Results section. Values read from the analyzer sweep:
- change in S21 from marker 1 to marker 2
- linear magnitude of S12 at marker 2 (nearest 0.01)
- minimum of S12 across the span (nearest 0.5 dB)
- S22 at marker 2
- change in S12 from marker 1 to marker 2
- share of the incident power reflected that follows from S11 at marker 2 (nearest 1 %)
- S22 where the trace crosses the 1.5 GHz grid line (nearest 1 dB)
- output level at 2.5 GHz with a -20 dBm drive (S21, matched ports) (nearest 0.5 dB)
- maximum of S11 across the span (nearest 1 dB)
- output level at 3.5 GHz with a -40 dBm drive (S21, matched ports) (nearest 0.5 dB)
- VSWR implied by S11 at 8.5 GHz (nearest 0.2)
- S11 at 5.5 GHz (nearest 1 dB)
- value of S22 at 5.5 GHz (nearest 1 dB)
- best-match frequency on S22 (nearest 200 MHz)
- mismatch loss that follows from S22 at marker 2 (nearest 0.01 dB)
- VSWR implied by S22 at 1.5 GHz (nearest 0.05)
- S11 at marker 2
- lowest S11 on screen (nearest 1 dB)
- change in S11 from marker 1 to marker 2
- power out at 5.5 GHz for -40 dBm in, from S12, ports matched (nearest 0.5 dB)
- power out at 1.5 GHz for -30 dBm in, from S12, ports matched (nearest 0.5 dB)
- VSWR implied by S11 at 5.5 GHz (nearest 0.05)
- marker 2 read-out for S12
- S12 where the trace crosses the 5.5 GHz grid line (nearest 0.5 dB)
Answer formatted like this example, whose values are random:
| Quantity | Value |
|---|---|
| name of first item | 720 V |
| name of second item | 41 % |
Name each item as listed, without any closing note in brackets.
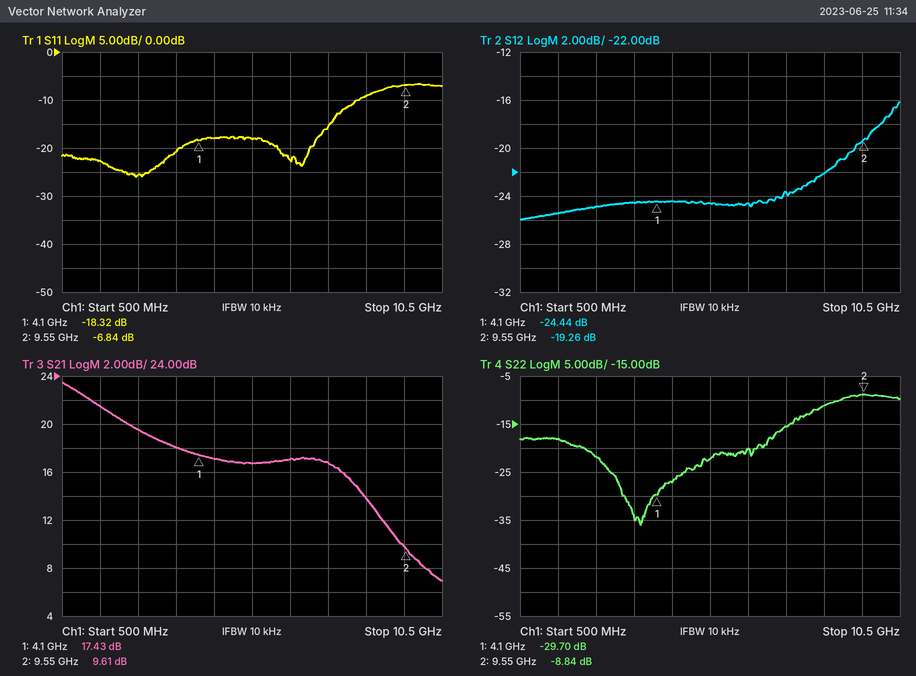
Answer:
| Quantity | Value |
|---|---|
| change in S21 from marker 1 to marker 2 | -7.82 dB |
| linear magnitude of S12 at marker 2 | 0.11 |
| minimum of S12 across the span | -26.0 dB |
| S22 at marker 2 | -8.84 dB |
| change in S12 from marker 1 to marker 2 | 5.18 dB |
| share of the incident power reflected that follows from S11 at marker 2 | 21 % |
| S22 where the trace crosses the 1.5 GHz grid line | -18 dB |
| output level at 2.5 GHz with a -20 dBm drive (S21, matched ports) | -0.5 dBm |
| maximum of S11 across the span | -7 dB |
| output level at 3.5 GHz with a -40 dBm drive (S21, matched ports) | -22.0 dBm |
| VSWR implied by S11 at 8.5 GHz | 2.0 |
| S11 at 5.5 GHz | -18 dB |
| value of S22 at 5.5 GHz | -22 dB |
| best-match frequency on S22 | 3.6 GHz |
| mismatch loss that follows from S22 at marker 2 | 0.61 dB |
| VSWR implied by S22 at 1.5 GHz | 1.30 |
| S11 at marker 2 | -6.84 dB |
| lowest S11 on screen | -26 dB |
| change in S11 from marker 1 to marker 2 | 11.48 dB |
| power out at 5.5 GHz for -40 dBm in, from S12, ports matched | -64.5 dBm |
| power out at 1.5 GHz for -30 dBm in, from S12, ports matched | -55.5 dBm |
| VSWR implied by S11 at 5.5 GHz | 1.30 |
| marker 2 read-out for S12 | -19.26 dB |
| S12 where the trace crosses the 5.5 GHz grid line | -24.5 dB |
